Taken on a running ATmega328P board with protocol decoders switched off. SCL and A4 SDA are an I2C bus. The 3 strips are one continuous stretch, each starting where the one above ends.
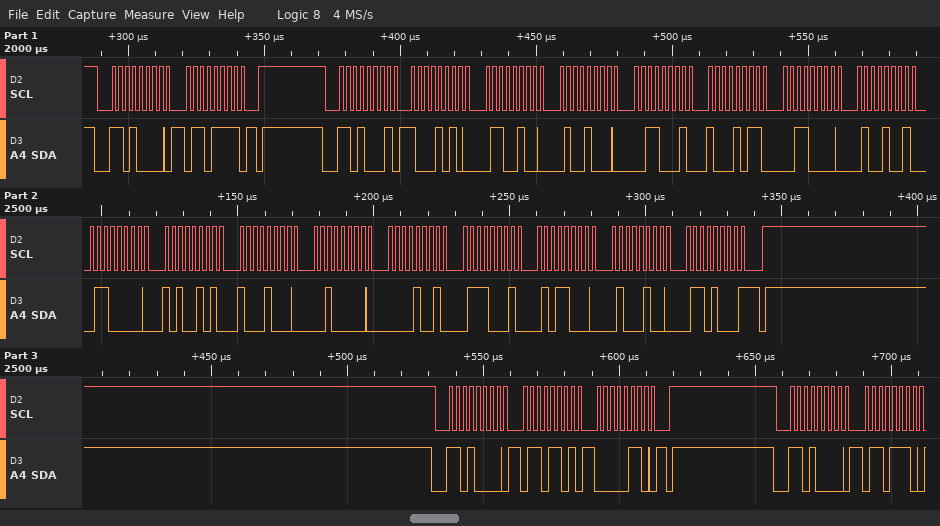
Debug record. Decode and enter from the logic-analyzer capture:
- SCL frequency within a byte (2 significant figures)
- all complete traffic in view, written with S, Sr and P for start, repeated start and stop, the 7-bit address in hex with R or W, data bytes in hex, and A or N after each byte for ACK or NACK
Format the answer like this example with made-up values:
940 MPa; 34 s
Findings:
400 kHz; S 68W A 6F A P S 68R A 8A A 64 A 48 A 31 A 8B A 30 A 49 A 60 A A5 A 88 A 20 A 09 A 71 A 58 A 44 A 68 N P S 68W A 6D A 06 A P S 68W A 6E A
